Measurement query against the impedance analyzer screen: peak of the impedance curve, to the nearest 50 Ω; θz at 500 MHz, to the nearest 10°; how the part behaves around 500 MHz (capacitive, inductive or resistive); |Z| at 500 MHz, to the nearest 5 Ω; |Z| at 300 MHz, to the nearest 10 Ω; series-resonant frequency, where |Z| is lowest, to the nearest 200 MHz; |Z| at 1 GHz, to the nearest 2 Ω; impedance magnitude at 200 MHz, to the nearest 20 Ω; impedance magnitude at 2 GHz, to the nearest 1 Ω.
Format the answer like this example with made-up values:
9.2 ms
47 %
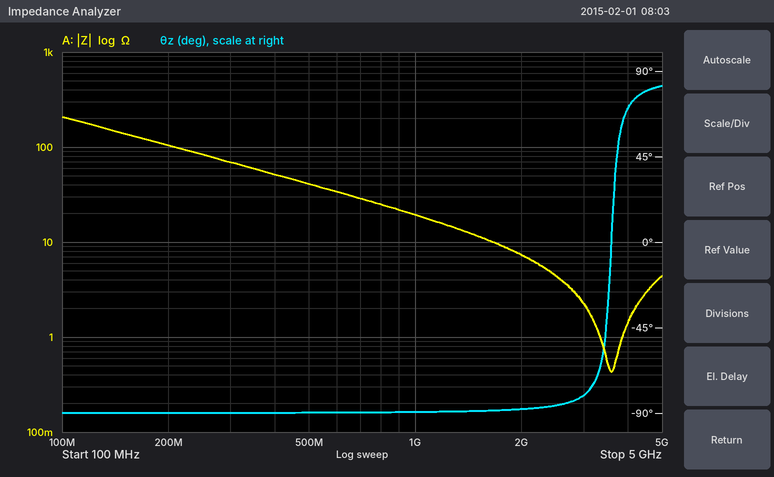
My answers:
200 Ω
-90°
capacitive
40 Ω
70 Ω
3.6 GHz
20 Ω
100 Ω
7 Ω
